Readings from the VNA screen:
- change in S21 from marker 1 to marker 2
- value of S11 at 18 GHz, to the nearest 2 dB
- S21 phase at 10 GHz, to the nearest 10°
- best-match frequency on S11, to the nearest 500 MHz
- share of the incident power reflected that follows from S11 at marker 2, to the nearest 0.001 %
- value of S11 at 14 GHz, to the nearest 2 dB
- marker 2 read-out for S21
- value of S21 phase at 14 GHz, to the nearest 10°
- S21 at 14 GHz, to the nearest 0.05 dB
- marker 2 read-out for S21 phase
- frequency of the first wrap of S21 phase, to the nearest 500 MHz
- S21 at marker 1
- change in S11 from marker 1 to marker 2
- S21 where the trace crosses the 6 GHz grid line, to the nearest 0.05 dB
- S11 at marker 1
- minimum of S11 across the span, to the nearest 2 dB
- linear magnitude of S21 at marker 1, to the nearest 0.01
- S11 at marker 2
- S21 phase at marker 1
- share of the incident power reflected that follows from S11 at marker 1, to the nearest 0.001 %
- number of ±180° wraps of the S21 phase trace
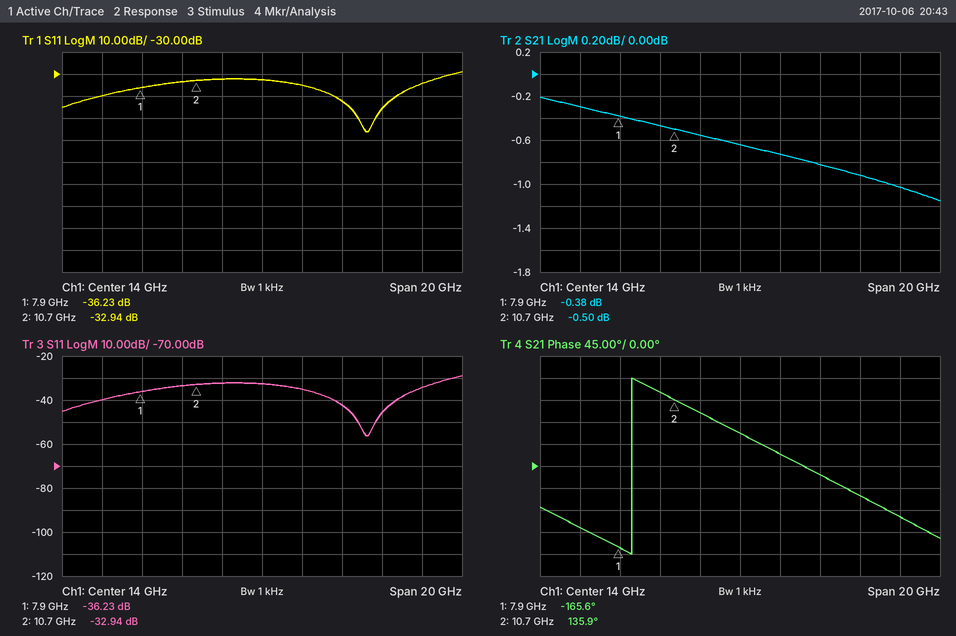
-0.12 dB
-42 dB
150°
19.0 GHz
0.051 %
-32 dB
-0.50 dB
70°
-0.65 dB
135.9°
8.5 GHz
-0.38 dB
3.29 dB
-0.30 dB
-36.23 dB
-56 dB
0.96
-32.94 dB
-165.6°
0.024 %
1
